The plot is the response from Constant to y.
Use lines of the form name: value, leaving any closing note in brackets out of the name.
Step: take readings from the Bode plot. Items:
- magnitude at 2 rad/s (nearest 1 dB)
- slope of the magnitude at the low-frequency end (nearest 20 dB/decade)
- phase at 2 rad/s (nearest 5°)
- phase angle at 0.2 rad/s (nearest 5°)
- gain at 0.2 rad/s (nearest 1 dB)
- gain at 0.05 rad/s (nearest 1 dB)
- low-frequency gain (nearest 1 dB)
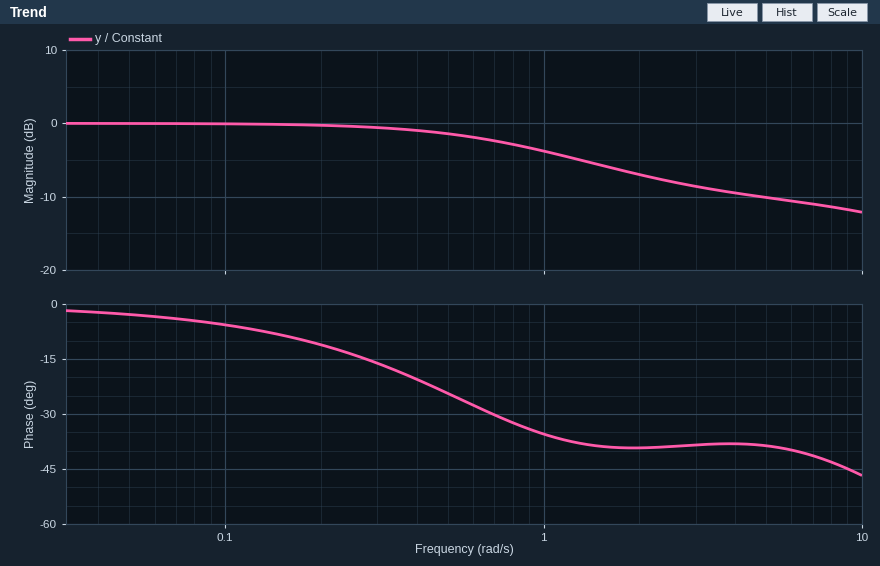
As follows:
magnitude at 2 rad/s: -7 dB
slope of the magnitude at the low-frequency end: 0 dB/decade
phase at 2 rad/s: -40°
phase angle at 0.2 rad/s: -10°
gain at 0.2 rad/s: 0 dB
gain at 0.05 rad/s: 0 dB
low-frequency gain: 0 dB
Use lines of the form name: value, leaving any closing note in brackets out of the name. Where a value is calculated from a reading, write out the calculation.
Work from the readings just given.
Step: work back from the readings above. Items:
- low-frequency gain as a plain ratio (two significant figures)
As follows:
low-frequency gain as a plain ratio: 10^(0 / 20) = 1.0
